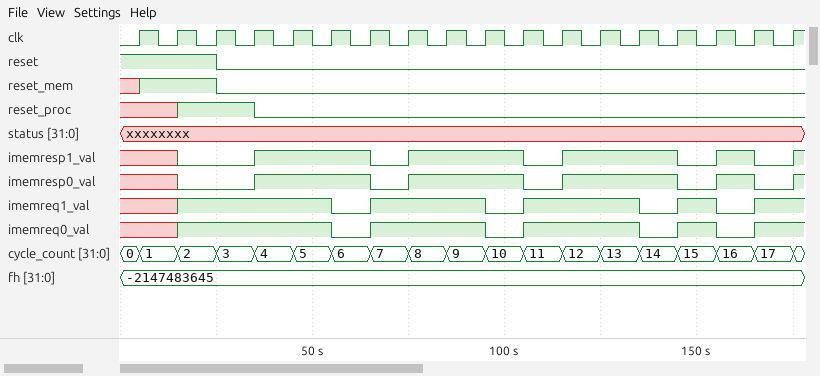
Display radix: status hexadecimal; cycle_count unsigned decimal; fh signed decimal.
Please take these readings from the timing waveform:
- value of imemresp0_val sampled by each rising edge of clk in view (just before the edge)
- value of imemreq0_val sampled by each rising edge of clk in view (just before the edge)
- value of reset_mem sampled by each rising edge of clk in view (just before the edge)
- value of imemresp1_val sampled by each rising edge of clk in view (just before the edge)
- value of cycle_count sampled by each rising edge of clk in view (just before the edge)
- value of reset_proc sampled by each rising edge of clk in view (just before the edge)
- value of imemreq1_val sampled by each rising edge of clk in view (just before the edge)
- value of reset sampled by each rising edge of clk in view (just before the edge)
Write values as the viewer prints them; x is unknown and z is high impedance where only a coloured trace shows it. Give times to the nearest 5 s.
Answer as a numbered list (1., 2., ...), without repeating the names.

1. x x 0 0 1 1 1 0 1 1 1 0 1 1 1 0 1 0
2. x x 1 1 1 1 0 1 1 1 0 1 1 1 0 1 0 1
3. x 1 1 0 0 0 0 0 0 0 0 0 0 0 0 0 0 0
4. x x 0 0 1 1 1 0 1 1 1 0 1 1 1 0 1 0
5. 0, 1, 2, 3, 4, 5, 6, 7, 8, 9, 10, 11, 12, 13, 14, 15, 16, 17
6. x x 1 1 0 0 0 0 0 0 0 0 0 0 0 0 0 0
7. x x 1 1 1 1 0 1 1 1 0 1 1 1 0 1 0 1
8. 1 1 1 0 0 0 0 0 0 0 0 0 0 0 0 0 0 0
